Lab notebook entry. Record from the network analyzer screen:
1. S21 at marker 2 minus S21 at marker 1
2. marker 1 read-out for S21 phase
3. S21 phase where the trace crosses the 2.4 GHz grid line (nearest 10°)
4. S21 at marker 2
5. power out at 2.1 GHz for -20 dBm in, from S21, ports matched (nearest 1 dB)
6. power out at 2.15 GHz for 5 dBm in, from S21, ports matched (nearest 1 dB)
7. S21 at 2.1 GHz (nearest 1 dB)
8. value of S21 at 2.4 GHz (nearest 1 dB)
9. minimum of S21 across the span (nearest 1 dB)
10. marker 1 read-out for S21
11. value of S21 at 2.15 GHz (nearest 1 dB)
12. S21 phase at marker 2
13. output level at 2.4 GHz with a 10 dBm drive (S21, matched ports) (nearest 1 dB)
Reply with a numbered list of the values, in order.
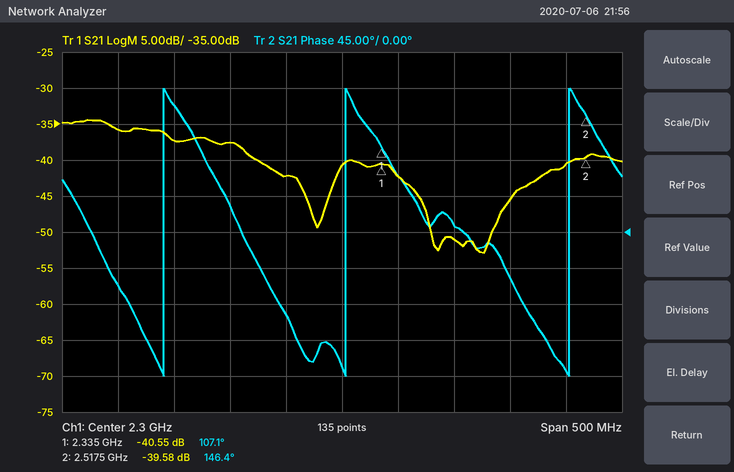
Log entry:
1. 0.97 dB
2. 107.1°
3. 10°
4. -39.58 dB
5. -56 dBm
6. -32 dBm
7. -36 dB
8. -51 dB
9. -53 dB
10. -40.55 dB
11. -37 dB
12. 146.4°
13. -41 dBm
